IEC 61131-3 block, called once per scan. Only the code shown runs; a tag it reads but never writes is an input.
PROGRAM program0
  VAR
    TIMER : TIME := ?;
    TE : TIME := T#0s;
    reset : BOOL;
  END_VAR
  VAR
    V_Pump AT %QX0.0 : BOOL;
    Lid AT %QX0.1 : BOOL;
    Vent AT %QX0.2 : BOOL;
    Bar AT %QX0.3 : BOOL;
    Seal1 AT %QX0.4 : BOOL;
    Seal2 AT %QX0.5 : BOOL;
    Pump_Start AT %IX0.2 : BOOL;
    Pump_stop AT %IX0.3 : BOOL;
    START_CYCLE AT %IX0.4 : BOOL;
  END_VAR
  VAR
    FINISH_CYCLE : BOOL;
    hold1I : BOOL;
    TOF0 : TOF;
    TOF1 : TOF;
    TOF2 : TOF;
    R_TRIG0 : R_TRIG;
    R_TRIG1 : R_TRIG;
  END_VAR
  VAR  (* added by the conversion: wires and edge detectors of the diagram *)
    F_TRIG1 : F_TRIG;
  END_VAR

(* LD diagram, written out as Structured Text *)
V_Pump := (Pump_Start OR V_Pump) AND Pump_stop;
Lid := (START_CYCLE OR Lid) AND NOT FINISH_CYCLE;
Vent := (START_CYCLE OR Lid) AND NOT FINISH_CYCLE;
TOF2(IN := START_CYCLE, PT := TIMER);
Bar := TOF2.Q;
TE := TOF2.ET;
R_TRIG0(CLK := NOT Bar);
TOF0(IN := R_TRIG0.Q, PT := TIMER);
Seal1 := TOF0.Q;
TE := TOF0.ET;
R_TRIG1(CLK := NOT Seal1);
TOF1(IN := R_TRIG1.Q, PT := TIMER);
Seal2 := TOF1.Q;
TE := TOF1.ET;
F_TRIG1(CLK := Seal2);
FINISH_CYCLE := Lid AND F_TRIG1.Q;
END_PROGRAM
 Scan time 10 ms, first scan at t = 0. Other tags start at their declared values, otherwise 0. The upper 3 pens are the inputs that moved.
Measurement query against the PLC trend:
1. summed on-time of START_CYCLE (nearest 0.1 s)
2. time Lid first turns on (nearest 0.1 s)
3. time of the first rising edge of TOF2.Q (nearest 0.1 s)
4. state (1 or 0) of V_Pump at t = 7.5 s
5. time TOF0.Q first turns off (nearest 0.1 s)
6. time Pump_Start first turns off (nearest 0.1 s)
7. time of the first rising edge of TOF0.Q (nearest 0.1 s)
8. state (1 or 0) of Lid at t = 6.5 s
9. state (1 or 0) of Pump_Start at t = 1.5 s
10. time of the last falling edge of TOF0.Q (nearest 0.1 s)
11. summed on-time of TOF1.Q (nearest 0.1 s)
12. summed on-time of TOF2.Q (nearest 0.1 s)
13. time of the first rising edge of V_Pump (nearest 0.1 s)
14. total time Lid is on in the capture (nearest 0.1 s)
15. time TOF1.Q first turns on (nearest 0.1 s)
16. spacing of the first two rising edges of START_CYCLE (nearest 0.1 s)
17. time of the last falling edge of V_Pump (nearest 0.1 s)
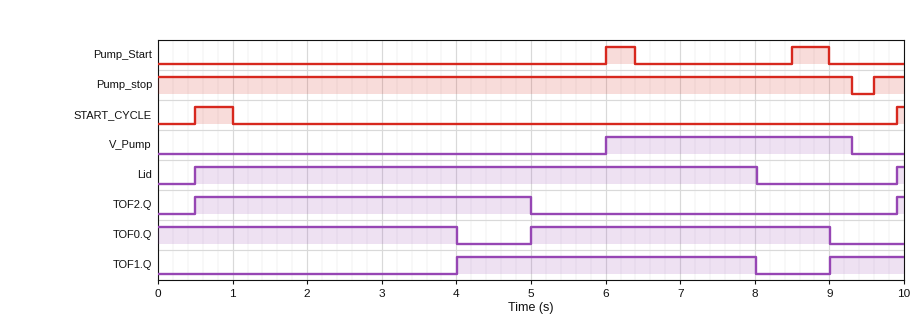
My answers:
0.6 s
0.5 s
0.5 s
1
4.0 s
6.4 s
5.0 s
1
0
9.0 s
5.0 s
4.6 s
6.0 s
7.6 s
4.0 s
9.4 s
9.3 s
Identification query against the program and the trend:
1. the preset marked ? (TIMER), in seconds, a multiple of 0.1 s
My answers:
4.0 s
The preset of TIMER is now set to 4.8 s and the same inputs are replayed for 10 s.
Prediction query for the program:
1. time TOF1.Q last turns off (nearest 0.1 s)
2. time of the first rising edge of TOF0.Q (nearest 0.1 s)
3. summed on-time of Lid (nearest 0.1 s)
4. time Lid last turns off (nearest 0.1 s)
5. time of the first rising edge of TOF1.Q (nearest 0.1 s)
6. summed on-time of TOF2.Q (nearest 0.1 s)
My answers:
9.6 s
5.8 s
9.2 s
9.6 s
4.8 s
5.4 s
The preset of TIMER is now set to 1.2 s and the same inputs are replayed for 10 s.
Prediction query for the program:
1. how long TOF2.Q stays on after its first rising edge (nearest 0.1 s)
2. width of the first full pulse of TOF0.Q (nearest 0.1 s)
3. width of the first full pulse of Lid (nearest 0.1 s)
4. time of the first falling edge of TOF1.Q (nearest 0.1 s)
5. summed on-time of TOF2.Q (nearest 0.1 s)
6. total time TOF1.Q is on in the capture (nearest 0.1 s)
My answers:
1.7 s
1.2 s
1.9 s
2.4 s
1.8 s
2.4 s
